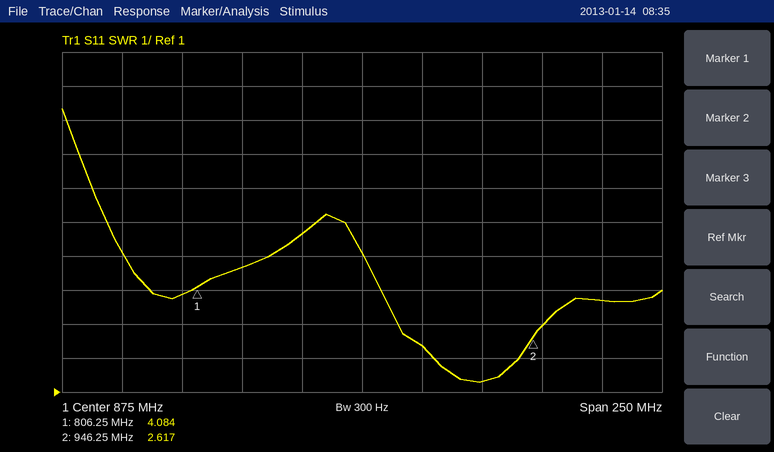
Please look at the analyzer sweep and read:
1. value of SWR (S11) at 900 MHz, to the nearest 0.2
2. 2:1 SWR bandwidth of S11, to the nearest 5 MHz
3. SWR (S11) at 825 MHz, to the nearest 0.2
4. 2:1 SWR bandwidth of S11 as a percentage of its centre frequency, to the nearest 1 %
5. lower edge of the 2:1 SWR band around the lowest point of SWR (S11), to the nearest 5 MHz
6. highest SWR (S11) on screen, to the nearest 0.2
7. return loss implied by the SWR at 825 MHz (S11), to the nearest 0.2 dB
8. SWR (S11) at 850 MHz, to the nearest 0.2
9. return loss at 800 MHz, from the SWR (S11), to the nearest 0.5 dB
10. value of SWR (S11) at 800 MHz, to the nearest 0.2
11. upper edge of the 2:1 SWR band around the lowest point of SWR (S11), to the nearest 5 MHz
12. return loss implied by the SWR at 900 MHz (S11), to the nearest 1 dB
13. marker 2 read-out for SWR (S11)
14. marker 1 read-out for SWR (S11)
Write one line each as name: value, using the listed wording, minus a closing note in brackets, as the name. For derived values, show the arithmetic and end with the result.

value of SWR (S11) at 900 MHz, to the nearest 0.2: 2.4
2:1 SWR bandwidth of S11, to the nearest 5 MHz: 940 MHz − 905 MHz = 35 MHz
SWR (S11) at 825 MHz, to the nearest 0.2: 4.6
2:1 SWR bandwidth of S11 as a percentage of its centre frequency, to the nearest 1 %: 35 MHz / 922.5 MHz ≈ 4 %
lower edge of the 2:1 SWR band around the lowest point of SWR (S11), to the nearest 5 MHz: 905 MHz
highest SWR (S11) on screen, to the nearest 0.2: 9.4
return loss implied by the SWR at 825 MHz (S11), to the nearest 0.2 dB: −20 log10((4.6 − 1)/(4.6 + 1)) ≈ 3.8 dB
SWR (S11) at 850 MHz, to the nearest 0.2: 5.6
return loss at 800 MHz, from the SWR (S11), to the nearest 0.5 dB: −20 log10((3.8 − 1)/(3.8 + 1)) ≈ 4.68 dB, so 4.5 dB to the nearest 0.5 dB
value of SWR (S11) at 800 MHz, to the nearest 0.2: 3.8
upper edge of the 2:1 SWR band around the lowest point of SWR (S11), to the nearest 5 MHz: 940 MHz
return loss implied by the SWR at 900 MHz (S11), to the nearest 1 dB: −20 log10((2.4 − 1)/(2.4 + 1)) ≈ 8 dB
marker 2 read-out for SWR: 2.617
marker 1 read-out for SWR: 4.084
